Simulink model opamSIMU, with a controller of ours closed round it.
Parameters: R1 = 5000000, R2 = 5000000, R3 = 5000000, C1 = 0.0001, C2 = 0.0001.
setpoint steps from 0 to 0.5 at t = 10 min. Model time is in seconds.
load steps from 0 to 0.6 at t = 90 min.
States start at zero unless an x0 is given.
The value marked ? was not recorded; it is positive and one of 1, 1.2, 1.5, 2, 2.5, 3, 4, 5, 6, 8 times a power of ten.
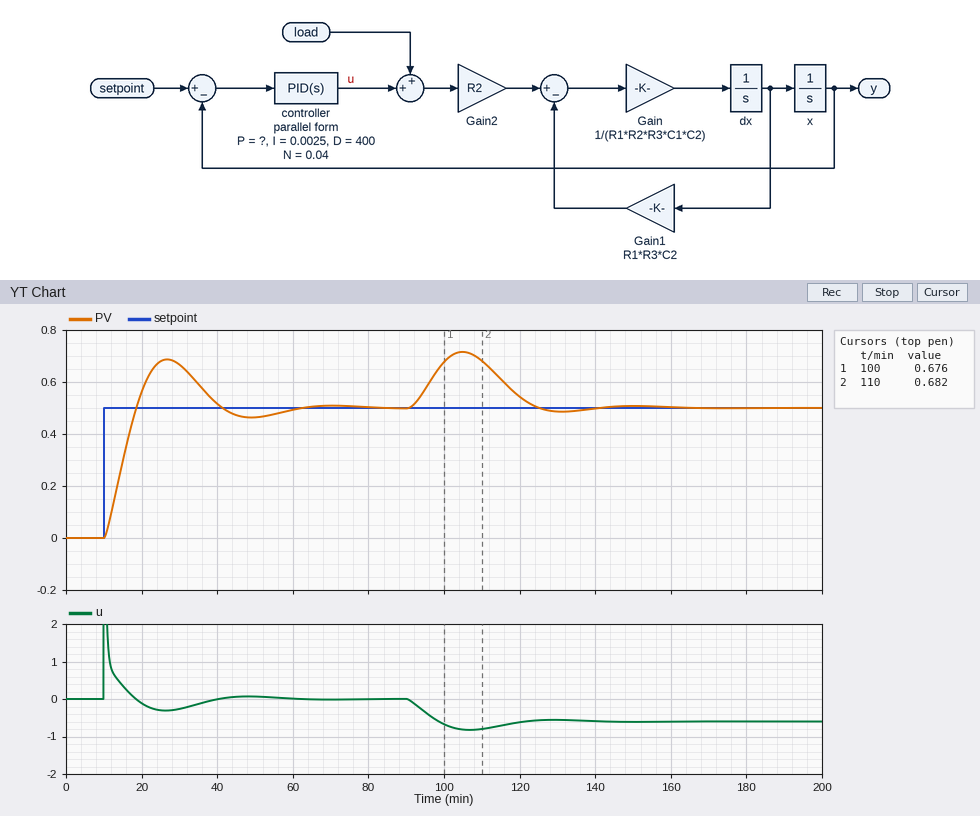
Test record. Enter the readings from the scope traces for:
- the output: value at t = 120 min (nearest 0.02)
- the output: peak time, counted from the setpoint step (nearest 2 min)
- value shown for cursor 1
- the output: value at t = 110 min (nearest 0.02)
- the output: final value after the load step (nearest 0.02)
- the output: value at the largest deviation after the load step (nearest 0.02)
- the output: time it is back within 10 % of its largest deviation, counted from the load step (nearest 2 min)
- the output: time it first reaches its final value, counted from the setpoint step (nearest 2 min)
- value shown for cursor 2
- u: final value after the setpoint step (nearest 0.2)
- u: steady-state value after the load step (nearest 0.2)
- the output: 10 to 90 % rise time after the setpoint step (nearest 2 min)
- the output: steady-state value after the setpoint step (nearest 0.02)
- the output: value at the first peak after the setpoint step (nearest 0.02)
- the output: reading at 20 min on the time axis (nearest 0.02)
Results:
0.54
16 min
0.676
0.68
0.50
0.72
32 min
8 min
0.682
0.0
-0.6
6 min
0.50
0.68
0.56
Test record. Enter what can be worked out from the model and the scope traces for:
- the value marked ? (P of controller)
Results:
2.5
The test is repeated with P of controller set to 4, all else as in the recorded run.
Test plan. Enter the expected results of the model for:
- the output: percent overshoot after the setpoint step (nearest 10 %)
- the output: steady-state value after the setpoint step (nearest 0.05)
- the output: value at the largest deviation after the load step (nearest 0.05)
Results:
40 %
0.50
0.65
